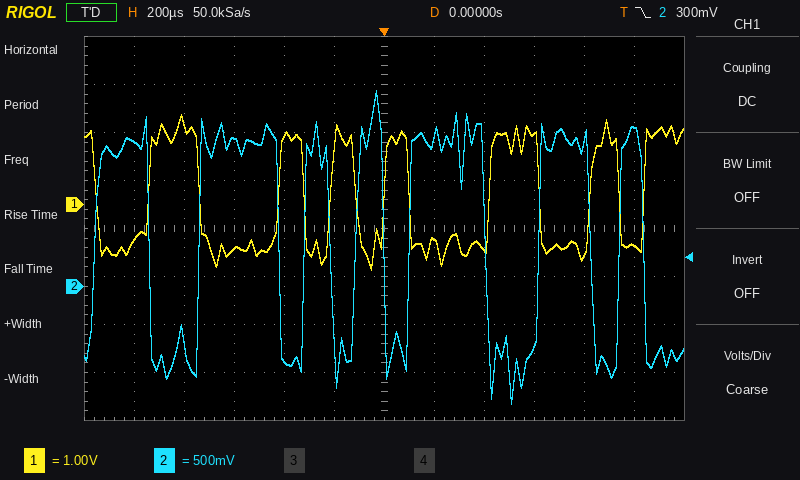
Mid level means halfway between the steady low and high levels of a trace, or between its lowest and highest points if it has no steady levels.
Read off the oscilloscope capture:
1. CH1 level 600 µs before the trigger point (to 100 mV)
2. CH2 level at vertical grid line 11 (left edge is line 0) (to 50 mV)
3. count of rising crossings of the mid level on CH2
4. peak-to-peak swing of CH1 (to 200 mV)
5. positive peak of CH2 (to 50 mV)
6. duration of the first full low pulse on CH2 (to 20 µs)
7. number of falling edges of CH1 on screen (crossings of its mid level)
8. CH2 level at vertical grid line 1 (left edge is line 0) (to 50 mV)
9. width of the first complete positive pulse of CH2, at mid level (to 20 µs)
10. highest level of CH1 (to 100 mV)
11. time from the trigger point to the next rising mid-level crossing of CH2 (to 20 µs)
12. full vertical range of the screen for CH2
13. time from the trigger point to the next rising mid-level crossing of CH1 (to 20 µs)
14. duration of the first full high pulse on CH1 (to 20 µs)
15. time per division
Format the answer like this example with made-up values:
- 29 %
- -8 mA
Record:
- -900 mV
- 1.65 V
- 7
- 3.2 V
- 2.05 V
- 200 µs
- 7
- 1.50 V
- 220 µs
- 1.9 V
- 100 µs
- 4 V
- 420 µs
- 200 µs
- 200 µs
